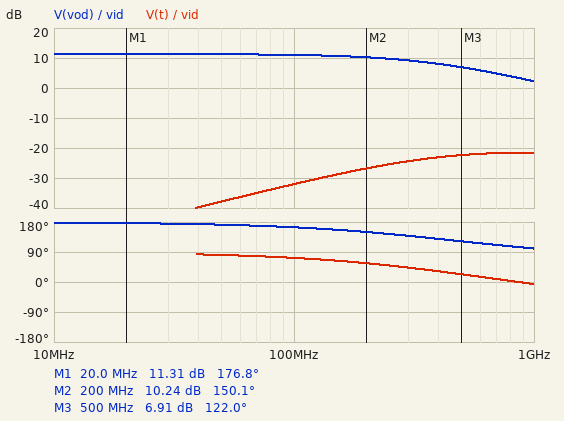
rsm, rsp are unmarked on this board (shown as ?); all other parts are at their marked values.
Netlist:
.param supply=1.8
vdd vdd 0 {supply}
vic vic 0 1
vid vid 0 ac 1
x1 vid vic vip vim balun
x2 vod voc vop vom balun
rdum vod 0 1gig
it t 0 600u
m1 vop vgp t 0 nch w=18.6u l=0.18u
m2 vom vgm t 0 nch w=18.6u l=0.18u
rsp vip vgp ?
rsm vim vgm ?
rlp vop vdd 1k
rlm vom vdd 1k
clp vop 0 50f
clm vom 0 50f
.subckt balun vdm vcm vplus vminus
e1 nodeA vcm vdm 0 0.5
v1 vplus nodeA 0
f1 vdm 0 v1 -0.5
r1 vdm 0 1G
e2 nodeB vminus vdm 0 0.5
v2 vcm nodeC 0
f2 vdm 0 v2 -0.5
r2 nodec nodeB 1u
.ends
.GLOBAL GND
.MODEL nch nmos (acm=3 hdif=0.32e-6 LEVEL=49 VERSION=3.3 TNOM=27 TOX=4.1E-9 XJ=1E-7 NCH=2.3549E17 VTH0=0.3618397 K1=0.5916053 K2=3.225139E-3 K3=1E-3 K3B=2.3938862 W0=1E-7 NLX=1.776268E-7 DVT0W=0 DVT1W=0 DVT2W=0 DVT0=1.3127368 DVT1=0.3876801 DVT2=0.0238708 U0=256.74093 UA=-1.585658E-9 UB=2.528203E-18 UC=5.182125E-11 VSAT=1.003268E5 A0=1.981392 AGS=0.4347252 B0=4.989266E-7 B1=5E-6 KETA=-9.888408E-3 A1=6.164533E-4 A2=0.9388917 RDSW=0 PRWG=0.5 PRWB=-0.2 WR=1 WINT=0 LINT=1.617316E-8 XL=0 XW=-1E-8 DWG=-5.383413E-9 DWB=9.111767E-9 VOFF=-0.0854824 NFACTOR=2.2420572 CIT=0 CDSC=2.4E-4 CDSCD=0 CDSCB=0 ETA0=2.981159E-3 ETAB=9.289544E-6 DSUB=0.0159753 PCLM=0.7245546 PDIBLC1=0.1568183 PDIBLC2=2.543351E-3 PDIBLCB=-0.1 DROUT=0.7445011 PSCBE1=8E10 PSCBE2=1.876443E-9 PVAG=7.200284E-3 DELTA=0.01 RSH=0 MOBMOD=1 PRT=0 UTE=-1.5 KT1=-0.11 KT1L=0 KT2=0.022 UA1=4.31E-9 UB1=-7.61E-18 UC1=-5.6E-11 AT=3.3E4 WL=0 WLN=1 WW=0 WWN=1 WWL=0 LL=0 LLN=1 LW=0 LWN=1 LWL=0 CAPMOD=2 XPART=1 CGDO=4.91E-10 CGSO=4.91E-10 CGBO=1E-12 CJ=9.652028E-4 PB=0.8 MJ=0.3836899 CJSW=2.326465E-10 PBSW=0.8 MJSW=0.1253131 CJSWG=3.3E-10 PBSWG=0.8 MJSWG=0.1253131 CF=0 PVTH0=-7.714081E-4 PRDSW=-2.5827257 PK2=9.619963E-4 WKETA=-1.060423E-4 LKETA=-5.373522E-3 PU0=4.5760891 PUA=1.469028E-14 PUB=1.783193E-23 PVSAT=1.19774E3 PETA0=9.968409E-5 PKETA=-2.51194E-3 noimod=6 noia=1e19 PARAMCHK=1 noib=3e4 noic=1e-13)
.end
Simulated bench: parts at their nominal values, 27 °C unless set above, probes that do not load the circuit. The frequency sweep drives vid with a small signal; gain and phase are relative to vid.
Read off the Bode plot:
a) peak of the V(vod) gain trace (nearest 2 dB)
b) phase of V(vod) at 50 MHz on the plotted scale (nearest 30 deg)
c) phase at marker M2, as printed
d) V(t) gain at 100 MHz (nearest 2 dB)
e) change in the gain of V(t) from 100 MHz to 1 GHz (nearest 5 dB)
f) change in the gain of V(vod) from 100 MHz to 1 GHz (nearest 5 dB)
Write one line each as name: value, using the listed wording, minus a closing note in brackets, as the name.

peak of the V(vod) gain trace: 12 dB
phase of V(vod) at 50 MHz on the plotted scale: 180 deg
phase at marker M2, as printed: 150.1 deg
V(t) gain at 100 MHz: -32 dB
change in the gain of V(t) from 100 MHz to 1 GHz: 10 dB
change in the gain of V(vod) from 100 MHz to 1 GHz: -10 dB
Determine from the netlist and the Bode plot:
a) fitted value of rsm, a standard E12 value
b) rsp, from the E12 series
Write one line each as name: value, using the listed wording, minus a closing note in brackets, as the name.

fitted value of rsm, a standard E12 value: 6.8 kΩ
rsp, from the E12 series: 3.9 kΩ
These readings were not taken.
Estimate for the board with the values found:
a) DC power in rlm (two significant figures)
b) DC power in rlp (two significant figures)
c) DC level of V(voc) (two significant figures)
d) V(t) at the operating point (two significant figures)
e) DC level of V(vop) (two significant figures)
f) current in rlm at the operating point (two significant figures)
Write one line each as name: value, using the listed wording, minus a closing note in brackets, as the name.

DC power in rlm: 90 µW
DC power in rlp: 90 µW
DC level of V(voc): 1.5 V
V(t) at the operating point: 320 mV
DC level of V(vop): 1.5 V
current in rlm at the operating point: 300 µA
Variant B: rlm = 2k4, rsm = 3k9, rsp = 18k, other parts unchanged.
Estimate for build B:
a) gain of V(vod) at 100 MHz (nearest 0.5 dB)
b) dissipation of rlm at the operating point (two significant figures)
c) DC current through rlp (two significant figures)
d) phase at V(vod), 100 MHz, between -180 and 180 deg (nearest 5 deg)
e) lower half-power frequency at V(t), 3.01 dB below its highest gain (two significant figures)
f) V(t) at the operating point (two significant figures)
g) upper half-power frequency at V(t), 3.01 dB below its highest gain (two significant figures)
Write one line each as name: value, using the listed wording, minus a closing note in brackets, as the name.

gain of V(vod) at 100 MHz: 14.0 dB
dissipation of rlm at the operating point: 190 µW
DC current through rlp: 320 µA
phase at V(vod), 100 MHz, between -180 and 180 deg: 150 deg
lower half-power frequency at V(t), 3.01 dB below its highest gain: 160 MHz
V(t) at the operating point: 310 mV
upper half-power frequency at V(t), 3.01 dB below its highest gain: 2.6 GHz
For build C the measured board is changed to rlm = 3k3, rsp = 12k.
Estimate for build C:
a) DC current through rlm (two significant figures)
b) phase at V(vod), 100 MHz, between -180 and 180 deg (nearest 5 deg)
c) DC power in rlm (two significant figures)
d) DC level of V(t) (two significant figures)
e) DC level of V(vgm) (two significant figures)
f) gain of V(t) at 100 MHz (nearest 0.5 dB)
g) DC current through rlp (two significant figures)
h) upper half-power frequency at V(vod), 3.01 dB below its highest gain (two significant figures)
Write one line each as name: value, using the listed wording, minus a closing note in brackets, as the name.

DC current through rlm: 270 µA
phase at V(vod), 100 MHz, between -180 and 180 deg: 145 deg
DC power in rlm: 240 µW
DC level of V(t): 310 mV
DC level of V(vgm): 1.0 V
gain of V(t) at 100 MHz: -23.5 dB
DC current through rlp: 330 µA
upper half-power frequency at V(vod), 3.01 dB below its highest gain: 170 MHz
